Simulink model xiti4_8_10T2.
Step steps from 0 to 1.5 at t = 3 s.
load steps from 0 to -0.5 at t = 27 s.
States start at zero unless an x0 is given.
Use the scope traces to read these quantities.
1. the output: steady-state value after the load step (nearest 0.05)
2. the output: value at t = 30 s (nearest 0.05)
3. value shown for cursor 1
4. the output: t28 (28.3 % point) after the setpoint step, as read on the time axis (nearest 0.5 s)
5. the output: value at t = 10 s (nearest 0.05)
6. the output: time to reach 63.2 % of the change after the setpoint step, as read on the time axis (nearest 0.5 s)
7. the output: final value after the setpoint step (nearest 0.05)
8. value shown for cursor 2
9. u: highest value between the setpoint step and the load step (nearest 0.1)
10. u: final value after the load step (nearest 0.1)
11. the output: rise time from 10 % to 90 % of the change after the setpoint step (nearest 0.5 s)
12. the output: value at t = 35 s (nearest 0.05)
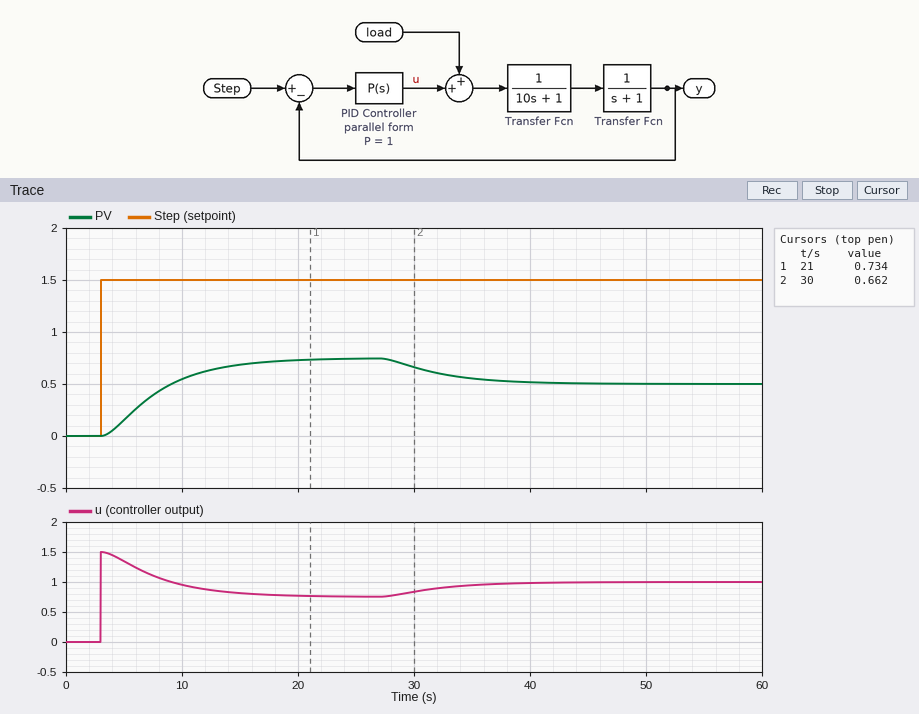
0.50
0.65
0.734
5.5 s
0.55
8.5 s
0.75
0.662
1.5
1.0
10.0 s
0.55
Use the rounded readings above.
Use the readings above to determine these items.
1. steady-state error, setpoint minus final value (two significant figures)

0.75
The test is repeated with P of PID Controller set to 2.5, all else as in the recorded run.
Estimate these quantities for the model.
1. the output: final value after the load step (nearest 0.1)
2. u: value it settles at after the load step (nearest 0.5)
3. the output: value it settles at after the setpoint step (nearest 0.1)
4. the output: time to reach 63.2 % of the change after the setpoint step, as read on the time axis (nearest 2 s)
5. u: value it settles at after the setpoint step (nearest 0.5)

0.9
1.5
1.1
6 s
1.0
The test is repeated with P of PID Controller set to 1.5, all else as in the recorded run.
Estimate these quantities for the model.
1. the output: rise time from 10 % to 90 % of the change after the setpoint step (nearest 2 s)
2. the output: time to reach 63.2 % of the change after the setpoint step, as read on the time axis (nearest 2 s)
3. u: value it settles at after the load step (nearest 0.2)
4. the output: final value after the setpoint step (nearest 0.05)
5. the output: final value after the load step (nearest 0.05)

8 s
8 s
1.2
0.90
0.70
